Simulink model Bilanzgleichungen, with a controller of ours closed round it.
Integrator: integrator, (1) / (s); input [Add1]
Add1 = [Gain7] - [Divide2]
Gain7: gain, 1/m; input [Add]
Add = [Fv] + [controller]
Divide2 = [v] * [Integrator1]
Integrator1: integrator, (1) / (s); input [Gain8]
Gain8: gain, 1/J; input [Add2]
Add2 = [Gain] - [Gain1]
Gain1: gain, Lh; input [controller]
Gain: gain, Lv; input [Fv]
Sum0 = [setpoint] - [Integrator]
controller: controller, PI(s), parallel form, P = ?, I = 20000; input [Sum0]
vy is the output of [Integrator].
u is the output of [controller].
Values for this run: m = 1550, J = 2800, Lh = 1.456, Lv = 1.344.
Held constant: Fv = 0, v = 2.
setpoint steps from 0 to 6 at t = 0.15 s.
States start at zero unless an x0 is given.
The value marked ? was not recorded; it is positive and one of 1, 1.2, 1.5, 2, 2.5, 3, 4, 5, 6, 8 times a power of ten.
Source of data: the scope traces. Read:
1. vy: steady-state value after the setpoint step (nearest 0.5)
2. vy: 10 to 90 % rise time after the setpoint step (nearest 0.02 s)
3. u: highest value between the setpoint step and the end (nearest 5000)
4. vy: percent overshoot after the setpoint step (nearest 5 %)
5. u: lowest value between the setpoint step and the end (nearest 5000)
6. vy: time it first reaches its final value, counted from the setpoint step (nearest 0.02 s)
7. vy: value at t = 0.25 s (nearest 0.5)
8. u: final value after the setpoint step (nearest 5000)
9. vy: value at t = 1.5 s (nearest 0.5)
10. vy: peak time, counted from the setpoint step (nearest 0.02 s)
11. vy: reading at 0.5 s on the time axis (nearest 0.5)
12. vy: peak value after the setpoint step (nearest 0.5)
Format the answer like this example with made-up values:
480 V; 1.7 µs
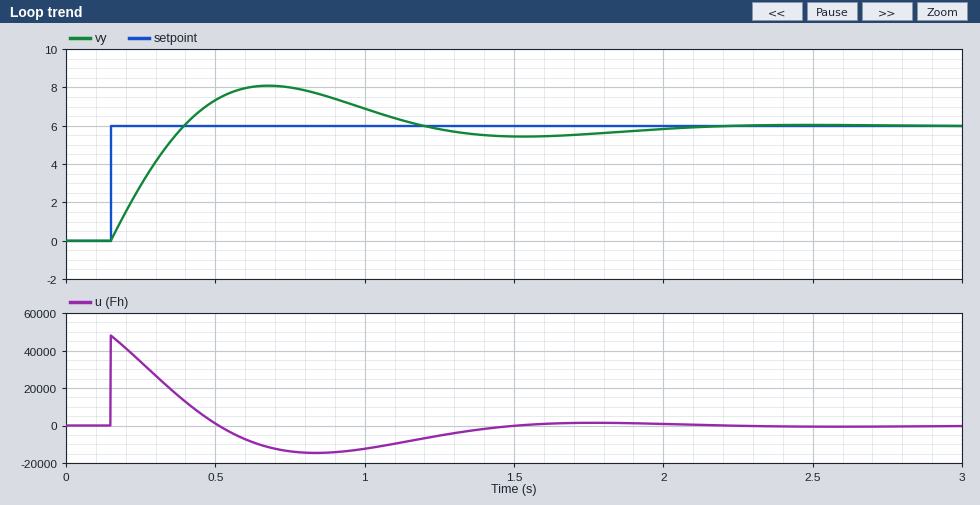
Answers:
6.0; 0.20 s; 50000; 35 %; -15000; 0.24 s; 3.0; 0; 5.5; 0.52 s; 7.5; 8.0
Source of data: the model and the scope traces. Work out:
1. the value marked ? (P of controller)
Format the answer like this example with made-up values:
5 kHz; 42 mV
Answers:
8000
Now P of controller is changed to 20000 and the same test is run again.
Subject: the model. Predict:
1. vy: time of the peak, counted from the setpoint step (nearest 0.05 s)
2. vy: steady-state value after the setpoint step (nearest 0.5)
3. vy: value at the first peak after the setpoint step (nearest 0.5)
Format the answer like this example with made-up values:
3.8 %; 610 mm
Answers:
0.35 s; 6.0; 7.0
